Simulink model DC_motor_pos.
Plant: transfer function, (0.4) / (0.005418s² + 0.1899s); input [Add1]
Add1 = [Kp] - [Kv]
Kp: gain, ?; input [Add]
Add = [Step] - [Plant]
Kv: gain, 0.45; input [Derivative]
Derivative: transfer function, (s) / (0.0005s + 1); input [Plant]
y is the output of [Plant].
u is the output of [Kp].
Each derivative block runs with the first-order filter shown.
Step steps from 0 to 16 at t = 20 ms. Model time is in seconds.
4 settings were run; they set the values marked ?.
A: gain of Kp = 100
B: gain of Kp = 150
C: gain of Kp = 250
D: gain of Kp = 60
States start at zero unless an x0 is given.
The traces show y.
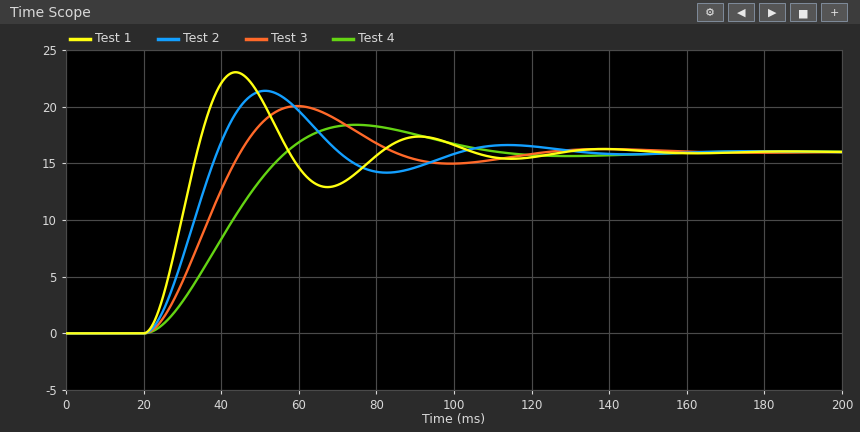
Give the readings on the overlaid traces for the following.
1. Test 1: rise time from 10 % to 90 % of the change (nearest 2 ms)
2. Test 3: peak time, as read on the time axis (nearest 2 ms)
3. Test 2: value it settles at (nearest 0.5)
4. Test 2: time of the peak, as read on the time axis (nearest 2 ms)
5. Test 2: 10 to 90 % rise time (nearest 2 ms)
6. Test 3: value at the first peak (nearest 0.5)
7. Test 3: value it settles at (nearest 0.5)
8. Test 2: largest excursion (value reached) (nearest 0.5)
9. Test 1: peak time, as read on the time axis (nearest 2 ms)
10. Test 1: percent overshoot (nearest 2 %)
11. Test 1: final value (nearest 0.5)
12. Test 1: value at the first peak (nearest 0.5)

10 ms
60 ms
16.0
52 ms
12 ms
20.0
16.0
21.5
44 ms
44 %
16.0
23.0
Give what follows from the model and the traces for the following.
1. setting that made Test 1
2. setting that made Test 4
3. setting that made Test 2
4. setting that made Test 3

C
D
B
A
